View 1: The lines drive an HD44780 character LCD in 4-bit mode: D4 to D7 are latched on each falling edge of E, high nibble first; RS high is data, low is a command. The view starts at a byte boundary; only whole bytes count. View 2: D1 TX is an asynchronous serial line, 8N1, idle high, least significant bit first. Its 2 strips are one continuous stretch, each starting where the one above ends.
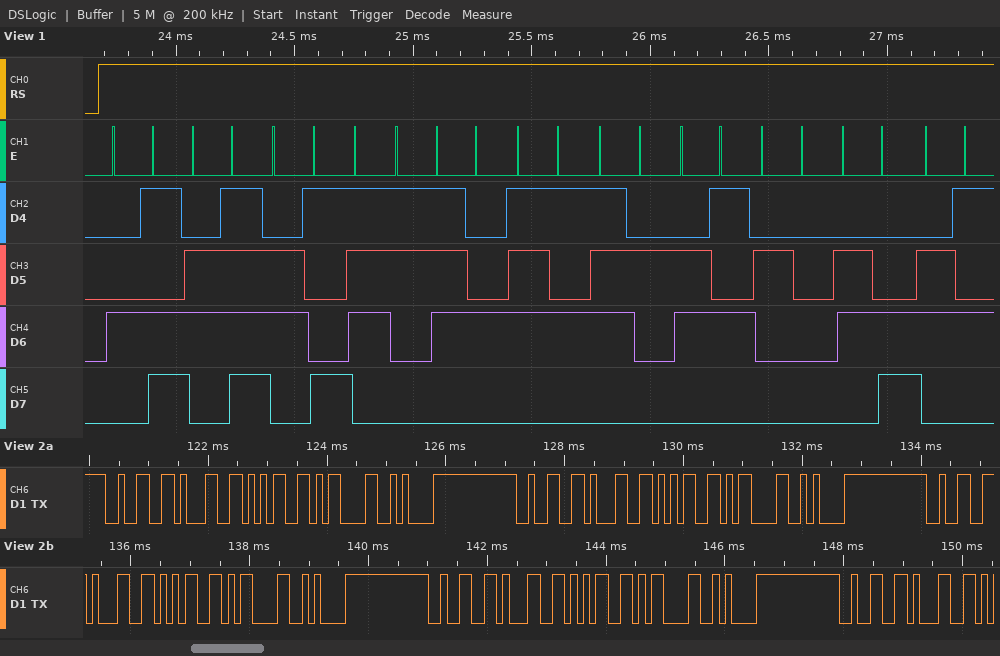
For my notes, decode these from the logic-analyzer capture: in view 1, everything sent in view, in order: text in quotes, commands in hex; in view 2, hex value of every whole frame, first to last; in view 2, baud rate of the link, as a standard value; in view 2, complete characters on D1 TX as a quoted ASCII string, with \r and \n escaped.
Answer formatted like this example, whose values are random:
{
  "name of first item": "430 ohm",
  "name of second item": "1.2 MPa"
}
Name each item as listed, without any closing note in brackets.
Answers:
{
  "in view 1, everything sent in view, in order: text in quotes, commands in hex": "\"Moisture le\"",
  "in view 2, hex value of every whole frame, first to last": "0x32 0x31 0x35 0x0D 0x0A 0x32 0x31 0x35 0x0D 0x0A 0x32 0x31 0x35 0x0D 0x0A 0x32 0x31 0x35 0x0D 0x0A 0x32 0x31",
  "in view 2, baud rate of the link, as a standard value": "9600 baud",
  "in view 2, complete characters on D1 TX as a quoted ASCII string, with \\r and \\n escaped": "\"215\\r\\n215\\r\\n215\\r\\n215\\r\\n21\""
}
